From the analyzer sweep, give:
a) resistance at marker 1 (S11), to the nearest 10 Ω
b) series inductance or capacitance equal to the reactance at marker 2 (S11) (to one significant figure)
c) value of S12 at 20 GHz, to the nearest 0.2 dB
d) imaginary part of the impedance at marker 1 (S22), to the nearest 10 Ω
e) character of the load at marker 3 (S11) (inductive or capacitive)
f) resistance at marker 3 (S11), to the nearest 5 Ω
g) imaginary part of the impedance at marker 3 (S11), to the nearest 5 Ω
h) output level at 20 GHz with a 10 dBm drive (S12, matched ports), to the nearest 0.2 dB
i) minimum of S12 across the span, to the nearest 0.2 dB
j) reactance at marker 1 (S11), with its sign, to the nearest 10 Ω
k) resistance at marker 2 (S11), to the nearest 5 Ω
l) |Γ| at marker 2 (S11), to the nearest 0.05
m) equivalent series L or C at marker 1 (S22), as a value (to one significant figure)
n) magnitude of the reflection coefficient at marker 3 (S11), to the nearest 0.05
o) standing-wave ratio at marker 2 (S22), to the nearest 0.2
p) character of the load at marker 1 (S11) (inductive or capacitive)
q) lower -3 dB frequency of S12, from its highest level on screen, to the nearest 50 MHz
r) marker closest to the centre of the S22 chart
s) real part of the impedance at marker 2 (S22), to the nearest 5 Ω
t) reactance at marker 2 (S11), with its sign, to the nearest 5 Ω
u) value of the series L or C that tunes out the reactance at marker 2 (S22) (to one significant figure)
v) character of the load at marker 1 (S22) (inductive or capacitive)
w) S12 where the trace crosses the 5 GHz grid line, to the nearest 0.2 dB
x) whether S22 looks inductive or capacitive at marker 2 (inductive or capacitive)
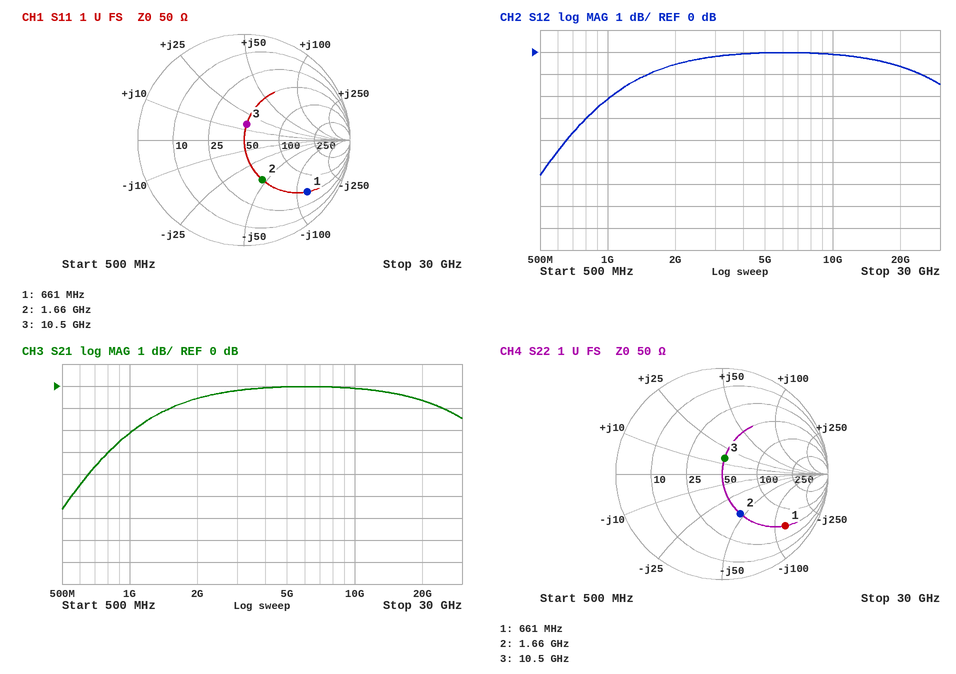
50 Ω
2 pF
-0.6 dB
-120 Ω
inductive
50 Ω
+15 Ω
9.4 dBm
-5.6 dB
-120 Ω
50 Ω
0.40
2 pF
0.15
2.4
capacitive
800 MHz
marker 3
50 Ω
-45 Ω
4 nH
capacitive
0.0 dB
capacitive
